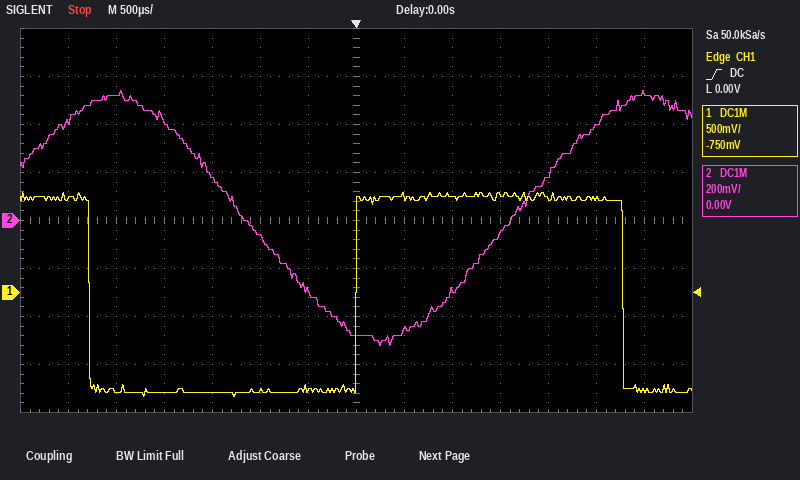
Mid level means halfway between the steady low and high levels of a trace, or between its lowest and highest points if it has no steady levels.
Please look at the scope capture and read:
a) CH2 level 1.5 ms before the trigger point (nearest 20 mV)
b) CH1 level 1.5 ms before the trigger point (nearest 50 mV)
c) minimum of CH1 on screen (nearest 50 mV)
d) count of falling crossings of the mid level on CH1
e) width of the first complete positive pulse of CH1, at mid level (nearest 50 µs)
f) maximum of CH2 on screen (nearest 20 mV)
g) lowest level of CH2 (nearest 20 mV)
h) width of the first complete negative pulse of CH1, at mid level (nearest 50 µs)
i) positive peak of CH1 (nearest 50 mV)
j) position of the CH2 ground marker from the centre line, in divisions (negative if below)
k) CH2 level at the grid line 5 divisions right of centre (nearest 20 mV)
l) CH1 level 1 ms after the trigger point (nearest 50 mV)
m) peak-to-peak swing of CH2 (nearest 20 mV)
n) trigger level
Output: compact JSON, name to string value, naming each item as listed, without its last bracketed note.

{"CH2 level 1.5 ms before the trigger point": "180 mV", "CH1 level 1.5 ms before the trigger point": "-1.05 V", "minimum of CH1 on screen": "-1.10 V", "count of falling crossings of the mid level on CH1": "2", "width of the first complete positive pulse of CH1, at mid level": "2.80 ms", "maximum of CH2 on screen": "540 mV", "lowest level of CH2": "-520 mV", "width of the first complete negative pulse of CH1, at mid level": "2.80 ms", "positive peak of CH1": "1.05 V", "position of the CH2 ground marker from the centre line, in divisions": "0.0 div", "CH2 level at the grid line 5 divisions right of centre": "400 mV", "CH1 level 1 ms after the trigger point": "1.00 V", "peak-to-peak swing of CH2": "1.06 V", "trigger level": "0.00 V"}
